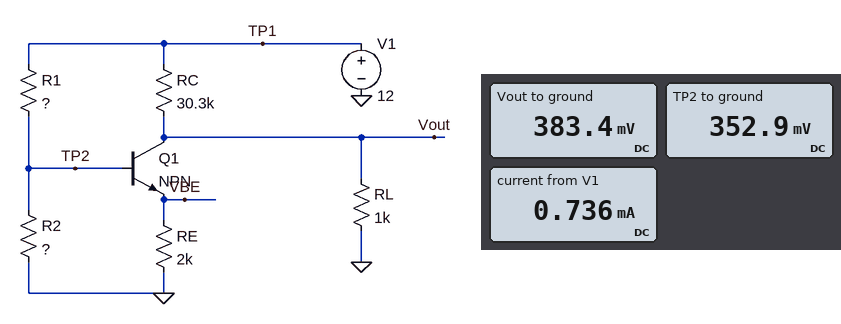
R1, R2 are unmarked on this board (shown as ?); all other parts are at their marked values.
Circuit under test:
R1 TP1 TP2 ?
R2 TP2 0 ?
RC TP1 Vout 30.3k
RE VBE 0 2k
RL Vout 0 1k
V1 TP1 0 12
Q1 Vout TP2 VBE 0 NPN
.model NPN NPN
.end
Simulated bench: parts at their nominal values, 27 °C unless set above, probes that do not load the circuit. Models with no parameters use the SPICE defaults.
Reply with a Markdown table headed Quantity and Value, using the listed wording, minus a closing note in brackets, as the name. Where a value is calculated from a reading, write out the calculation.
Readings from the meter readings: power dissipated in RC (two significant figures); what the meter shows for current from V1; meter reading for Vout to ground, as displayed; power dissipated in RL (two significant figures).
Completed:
| Quantity | Value |
|---|---|
| power dissipated in RC | (12 V - 383.4 mV)^2 / 30.3 kΩ = 4.5 mW |
| what the meter shows for current from V1 | 0.736 mA |
| meter reading for Vout to ground, as displayed | 383.4 mV |
| power dissipated in RL | (383.4 mV)^2 / 1 kΩ = 150 µW |
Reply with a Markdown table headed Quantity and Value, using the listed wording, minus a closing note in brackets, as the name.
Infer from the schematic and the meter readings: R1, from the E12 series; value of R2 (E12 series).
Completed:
| Quantity | Value |
|---|---|
| R1, from the E12 series | 33 kΩ |
| value of R2 | 1 kΩ |
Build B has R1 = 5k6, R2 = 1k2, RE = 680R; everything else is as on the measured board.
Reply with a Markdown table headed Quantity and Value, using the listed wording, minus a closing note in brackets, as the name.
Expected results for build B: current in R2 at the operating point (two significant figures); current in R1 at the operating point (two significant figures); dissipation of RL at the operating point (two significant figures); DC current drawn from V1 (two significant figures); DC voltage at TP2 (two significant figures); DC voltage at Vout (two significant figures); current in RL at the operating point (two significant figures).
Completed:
| Quantity | Value |
|---|---|
| current in R2 at the operating point | 1.1 mA |
| current in R1 at the operating point | 1.9 mA |
| dissipation of RL at the operating point | 260 µW |
| DC current drawn from V1 | 2.3 mA |
| DC voltage at TP2 | 1.3 V |
| DC voltage at Vout | 510 mV |
| current in RL at the operating point | 510 µA |
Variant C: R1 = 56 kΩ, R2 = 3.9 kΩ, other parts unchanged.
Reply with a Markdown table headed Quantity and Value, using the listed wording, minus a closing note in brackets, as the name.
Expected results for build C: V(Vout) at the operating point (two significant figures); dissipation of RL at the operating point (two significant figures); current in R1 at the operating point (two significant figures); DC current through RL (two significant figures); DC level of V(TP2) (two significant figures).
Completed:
| Quantity | Value |
|---|---|
| V(Vout) at the operating point | 340 mV |
| dissipation of RL at the operating point | 120 µW |
| current in R1 at the operating point | 200 µA |
| DC current through RL | 340 µA |
| DC level of V(TP2) | 780 mV |
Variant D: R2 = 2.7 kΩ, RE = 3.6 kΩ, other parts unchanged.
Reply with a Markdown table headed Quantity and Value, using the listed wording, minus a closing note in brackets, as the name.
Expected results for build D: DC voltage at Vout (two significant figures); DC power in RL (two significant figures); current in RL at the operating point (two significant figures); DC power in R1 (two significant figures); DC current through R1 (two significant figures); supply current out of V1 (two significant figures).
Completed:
| Quantity | Value |
|---|---|
| DC voltage at Vout | 330 mV |
| DC power in RL | 110 µW |
| current in RL at the operating point | 330 µA |
| DC power in R1 | 3.7 mW |
| DC current through R1 | 340 µA |
| supply current out of V1 | 720 µA |
